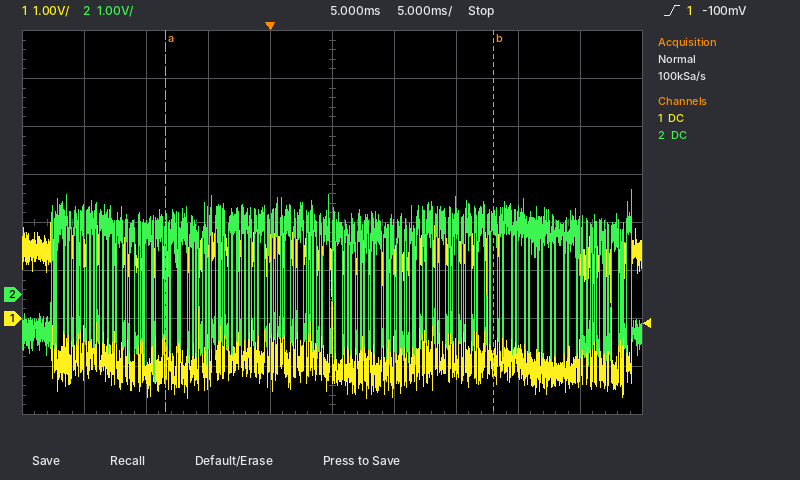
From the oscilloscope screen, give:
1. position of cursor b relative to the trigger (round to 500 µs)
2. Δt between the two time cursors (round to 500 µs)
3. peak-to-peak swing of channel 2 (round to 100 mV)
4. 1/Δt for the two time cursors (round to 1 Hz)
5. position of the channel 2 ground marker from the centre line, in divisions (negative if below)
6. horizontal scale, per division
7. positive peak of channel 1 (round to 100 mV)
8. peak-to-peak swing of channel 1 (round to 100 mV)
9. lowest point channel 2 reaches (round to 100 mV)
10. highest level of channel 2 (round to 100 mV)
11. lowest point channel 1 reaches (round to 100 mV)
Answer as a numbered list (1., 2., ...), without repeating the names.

1. +18.0 ms
2. 26.5 ms
3. 4.0 V
4. 38 Hz
5. -1.5 div
6. 5 ms
7. 2.0 V
8. 3.7 V
9. -1.8 V
10. 2.2 V
11. -1.7 V
